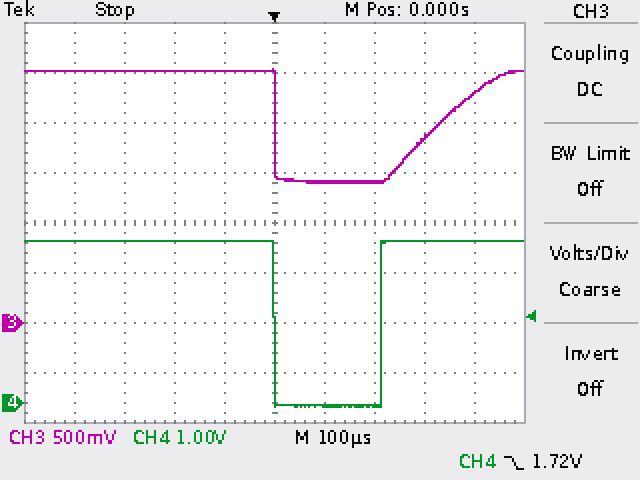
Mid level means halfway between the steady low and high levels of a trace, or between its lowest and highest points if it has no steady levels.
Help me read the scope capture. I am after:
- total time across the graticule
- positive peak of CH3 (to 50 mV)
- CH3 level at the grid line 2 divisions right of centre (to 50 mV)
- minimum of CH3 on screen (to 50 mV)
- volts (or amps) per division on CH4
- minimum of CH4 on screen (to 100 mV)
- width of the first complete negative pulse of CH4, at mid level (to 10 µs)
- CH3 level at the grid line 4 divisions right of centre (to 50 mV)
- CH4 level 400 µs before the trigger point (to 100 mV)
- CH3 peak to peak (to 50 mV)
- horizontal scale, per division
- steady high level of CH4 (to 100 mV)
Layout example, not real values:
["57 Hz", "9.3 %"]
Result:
["1 ms", "2.55 V", "1.40 V", "1.40 V", "1 V", "-100 mV", "210 µs", "2.30 V", "3.2 V", "1.15 V", "100 µs", "3.2 V"]
